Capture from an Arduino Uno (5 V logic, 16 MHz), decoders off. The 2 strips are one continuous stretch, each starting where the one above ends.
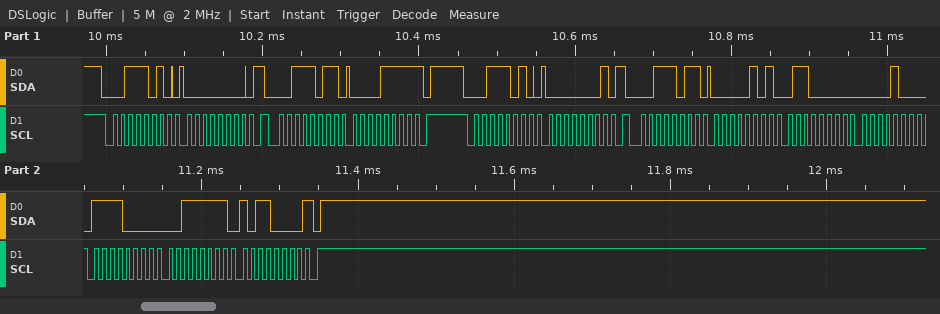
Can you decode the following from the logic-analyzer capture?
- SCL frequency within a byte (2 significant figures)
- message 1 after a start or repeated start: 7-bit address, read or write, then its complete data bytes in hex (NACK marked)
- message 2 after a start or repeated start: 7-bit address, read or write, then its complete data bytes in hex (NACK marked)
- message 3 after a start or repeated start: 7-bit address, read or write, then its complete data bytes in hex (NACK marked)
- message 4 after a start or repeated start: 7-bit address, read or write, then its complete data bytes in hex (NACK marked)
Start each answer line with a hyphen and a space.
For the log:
- 100 kHz
- 0x1D write: 00
- 0x1D read: 0F NACK
- 0x1D write: 01
- 0x1D read: 05 60 08 F0 3F B0 NACK
